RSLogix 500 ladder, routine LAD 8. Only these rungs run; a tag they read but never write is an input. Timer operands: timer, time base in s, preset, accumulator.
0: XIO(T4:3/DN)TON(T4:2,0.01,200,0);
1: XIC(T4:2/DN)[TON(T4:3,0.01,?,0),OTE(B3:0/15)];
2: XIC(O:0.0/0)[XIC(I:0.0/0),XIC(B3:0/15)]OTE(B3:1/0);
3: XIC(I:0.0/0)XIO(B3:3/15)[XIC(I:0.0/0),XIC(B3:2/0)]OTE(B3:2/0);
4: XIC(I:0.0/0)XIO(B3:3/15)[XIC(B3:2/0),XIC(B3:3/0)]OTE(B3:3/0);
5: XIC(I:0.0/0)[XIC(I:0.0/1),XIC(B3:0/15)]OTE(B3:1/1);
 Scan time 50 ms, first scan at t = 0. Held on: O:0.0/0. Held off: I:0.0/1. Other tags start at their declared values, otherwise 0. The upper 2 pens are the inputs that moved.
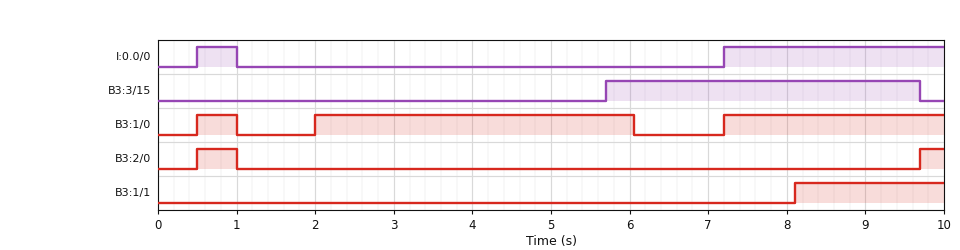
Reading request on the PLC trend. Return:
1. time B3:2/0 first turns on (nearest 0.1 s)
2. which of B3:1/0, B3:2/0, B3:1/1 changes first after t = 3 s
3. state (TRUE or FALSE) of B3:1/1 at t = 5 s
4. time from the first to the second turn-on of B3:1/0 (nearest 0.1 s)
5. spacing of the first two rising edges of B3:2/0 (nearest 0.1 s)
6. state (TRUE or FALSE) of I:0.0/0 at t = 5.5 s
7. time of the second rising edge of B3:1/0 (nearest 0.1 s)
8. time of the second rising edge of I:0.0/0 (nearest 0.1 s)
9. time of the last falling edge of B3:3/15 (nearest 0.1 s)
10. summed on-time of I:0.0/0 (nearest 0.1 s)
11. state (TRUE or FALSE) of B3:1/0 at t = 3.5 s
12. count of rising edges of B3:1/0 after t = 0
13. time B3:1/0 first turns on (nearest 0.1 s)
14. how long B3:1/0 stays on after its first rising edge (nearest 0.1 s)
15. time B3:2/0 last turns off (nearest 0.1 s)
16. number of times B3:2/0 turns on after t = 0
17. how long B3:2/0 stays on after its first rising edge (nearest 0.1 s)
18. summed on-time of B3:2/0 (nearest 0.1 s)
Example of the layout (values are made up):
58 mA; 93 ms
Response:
0.5 s; B3:1/0; FALSE; 1.5 s; 9.2 s; FALSE; 2.0 s; 7.2 s; 9.7 s; 3.3 s; TRUE; 3; 0.5 s; 0.5 s; 1.0 s; 2; 0.5 s; 0.8 s
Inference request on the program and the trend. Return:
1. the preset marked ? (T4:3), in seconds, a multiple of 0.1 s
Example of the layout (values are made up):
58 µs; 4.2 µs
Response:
4.0 s
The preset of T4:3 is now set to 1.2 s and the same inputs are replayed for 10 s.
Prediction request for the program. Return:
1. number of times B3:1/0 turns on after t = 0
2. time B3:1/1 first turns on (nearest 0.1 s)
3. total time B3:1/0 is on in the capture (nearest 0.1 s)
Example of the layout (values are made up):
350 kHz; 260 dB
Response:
4; 8.6 s; 5.8 s
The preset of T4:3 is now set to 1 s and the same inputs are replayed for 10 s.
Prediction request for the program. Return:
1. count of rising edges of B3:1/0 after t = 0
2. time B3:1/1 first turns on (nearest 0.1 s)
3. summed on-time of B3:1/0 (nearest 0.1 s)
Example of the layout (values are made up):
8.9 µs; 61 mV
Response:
4; 8.2 s; 5.4 s
